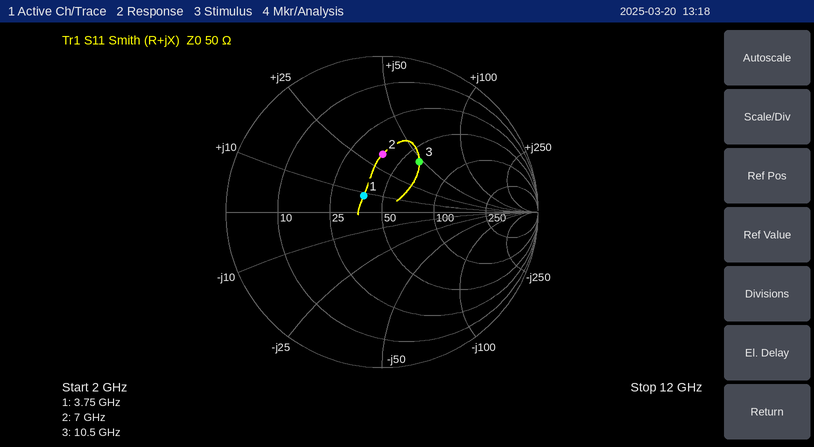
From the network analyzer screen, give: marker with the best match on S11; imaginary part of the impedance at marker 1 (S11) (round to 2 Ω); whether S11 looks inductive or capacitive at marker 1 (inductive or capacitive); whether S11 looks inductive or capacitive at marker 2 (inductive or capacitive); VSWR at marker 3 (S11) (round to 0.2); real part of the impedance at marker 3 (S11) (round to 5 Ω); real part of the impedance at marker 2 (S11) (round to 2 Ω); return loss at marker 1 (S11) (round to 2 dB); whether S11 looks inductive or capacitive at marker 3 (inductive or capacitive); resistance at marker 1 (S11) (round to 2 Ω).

marker 1
+8 Ω
inductive
inductive
2.4
60 Ω
38 Ω
16 dB
inductive
38 Ω
